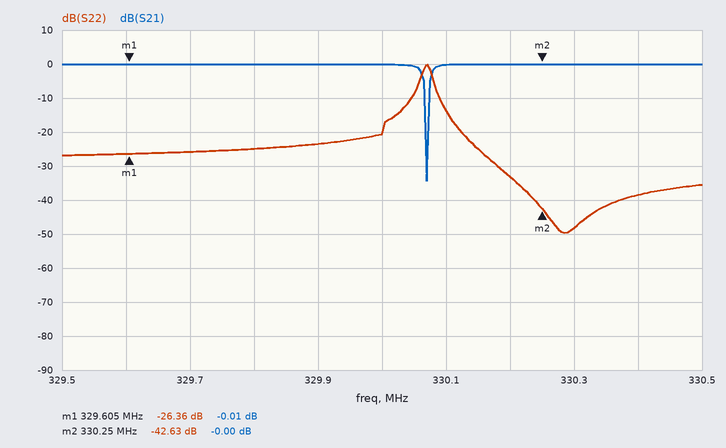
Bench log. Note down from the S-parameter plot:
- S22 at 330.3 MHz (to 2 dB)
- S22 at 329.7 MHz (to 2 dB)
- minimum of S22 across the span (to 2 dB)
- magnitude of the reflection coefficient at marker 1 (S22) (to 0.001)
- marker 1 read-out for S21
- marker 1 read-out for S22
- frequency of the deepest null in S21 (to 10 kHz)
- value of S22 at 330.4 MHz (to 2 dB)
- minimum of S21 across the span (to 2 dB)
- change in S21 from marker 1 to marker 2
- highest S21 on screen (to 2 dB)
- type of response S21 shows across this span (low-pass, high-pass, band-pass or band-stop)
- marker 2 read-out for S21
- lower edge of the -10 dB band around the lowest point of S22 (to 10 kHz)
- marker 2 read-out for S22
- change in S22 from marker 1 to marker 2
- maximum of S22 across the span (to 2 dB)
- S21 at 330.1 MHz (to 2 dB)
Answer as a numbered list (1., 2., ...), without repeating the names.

1. -48 dB
2. -26 dB
3. -50 dB
4. 0.048
5. -0.01 dB
6. -26.36 dB
7. 330.07 MHz
8. -38 dB
9. -34 dB
10. 0.01 dB
11. 0 dB
12. band-stop
13. -0.00 dB
14. 330.09 MHz
15. -42.63 dB
16. -16.27 dB
17. 0 dB
18. 0 dB
